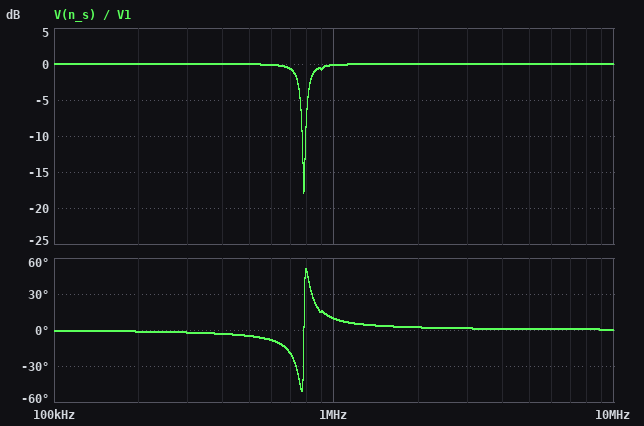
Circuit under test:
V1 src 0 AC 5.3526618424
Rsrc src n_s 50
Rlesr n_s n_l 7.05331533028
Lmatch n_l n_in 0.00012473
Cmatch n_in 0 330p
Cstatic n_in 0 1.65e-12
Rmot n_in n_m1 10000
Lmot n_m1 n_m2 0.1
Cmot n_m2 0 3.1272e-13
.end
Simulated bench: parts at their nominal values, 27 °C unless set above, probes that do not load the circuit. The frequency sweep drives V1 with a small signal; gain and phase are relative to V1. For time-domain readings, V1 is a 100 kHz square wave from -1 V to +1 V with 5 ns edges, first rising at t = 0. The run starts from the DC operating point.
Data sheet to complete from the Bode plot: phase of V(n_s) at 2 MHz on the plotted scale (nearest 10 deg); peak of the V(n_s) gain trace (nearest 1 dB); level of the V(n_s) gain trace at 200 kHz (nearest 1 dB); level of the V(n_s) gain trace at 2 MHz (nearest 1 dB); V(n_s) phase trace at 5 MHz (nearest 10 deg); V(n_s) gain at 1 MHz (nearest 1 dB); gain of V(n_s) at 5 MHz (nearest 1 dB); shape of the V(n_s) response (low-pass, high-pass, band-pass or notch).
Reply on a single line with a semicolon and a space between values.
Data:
0 deg; 0 dB; 0 dB; 0 dB; 0 deg; 0 dB; 0 dB; notch
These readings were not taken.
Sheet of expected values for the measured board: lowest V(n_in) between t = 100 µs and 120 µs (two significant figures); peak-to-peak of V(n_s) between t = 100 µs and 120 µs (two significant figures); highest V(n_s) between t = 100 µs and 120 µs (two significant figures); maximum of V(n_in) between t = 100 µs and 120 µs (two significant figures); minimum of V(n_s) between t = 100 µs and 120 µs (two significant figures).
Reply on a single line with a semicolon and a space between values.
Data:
-2.4 V; 2.2 V; 1.1 V; 2.4 V; -1.1 V
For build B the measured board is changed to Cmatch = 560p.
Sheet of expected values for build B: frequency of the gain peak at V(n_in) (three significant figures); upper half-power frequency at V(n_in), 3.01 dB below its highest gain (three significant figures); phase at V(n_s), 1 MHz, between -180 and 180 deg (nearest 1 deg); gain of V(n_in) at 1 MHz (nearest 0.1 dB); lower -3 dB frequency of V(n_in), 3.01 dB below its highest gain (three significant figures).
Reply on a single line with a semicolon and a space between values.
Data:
599 kHz; 634 kHz; 6 deg; -5.0 dB; 561 kHz
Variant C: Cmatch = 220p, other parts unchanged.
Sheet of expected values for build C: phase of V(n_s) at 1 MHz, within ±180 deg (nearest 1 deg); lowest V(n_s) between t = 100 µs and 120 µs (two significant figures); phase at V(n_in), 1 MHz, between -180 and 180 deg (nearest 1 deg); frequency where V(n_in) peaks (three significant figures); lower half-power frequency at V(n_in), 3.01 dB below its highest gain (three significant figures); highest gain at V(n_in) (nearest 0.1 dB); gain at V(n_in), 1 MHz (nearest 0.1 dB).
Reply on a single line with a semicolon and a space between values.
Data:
36 deg; -1.1 V; -137 deg; 961 kHz; 929 kHz; 22.3 dB; 18.7 dB
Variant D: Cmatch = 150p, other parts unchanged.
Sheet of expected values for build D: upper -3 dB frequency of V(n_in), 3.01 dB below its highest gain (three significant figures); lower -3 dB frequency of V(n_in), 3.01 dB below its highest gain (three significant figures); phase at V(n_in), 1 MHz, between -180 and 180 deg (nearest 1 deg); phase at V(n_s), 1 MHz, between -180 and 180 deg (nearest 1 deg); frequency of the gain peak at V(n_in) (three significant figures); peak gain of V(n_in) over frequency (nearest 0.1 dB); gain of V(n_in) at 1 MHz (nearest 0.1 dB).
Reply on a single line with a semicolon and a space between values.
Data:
1.19 MHz; 1.12 MHz; -12 deg; -10 deg; 1.16 MHz; 24.0 dB; 11.5 dB
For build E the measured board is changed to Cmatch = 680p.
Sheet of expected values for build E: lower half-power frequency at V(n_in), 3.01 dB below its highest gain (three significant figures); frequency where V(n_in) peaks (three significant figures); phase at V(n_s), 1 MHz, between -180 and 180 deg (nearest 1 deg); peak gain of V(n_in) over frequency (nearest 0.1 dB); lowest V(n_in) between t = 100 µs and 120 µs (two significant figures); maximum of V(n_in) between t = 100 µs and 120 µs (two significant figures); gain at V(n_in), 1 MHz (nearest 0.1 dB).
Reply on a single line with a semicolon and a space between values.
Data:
505 kHz; 543 kHz; 5 deg; 17.5 dB; -2.7 V; 2.7 V; -7.5 dB
